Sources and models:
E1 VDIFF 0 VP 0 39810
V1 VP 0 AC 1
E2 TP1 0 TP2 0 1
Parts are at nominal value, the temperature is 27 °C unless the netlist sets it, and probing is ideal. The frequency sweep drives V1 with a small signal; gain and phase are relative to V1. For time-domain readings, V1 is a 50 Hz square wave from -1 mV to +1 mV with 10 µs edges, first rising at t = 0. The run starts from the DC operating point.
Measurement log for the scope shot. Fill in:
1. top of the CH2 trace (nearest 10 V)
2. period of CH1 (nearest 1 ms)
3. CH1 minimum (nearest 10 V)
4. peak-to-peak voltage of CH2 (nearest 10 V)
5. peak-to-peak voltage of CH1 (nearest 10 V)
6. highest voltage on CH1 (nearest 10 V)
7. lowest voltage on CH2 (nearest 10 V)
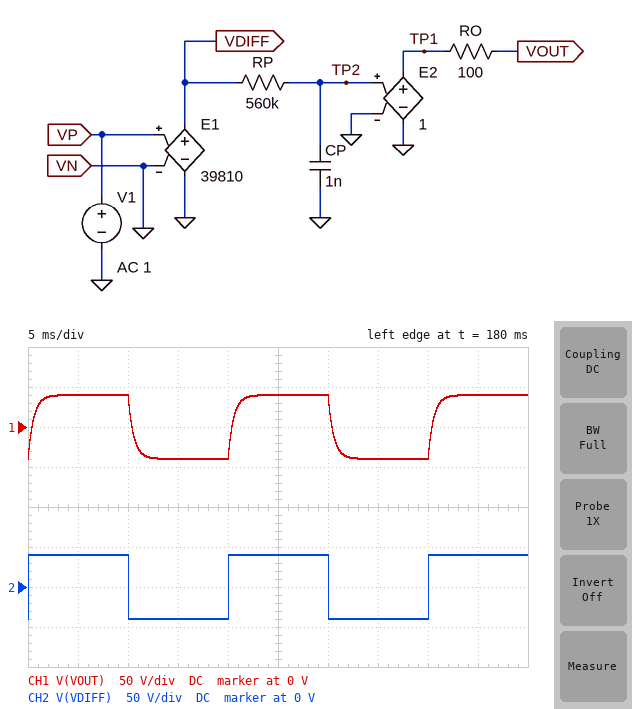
40 V
20 ms
-40 V
80 V
80 V
40 V
-40 V
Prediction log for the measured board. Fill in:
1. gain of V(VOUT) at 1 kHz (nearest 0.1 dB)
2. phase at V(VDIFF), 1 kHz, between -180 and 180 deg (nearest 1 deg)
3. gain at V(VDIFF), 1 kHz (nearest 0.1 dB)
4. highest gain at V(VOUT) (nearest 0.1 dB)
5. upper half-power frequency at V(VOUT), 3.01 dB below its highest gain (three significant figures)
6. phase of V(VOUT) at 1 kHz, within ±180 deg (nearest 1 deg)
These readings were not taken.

80.7 dB
0 deg
92.0 dB
92.0 dB
284 Hz
-74 deg
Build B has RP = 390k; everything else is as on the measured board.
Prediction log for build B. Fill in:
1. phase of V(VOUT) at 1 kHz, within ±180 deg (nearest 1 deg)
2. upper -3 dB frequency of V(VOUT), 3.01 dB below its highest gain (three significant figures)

-68 deg
408 Hz
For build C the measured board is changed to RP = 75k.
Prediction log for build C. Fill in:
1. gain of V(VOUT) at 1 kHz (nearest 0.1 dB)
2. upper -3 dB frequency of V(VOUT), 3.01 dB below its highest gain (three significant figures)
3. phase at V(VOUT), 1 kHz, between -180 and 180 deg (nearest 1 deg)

91.1 dB
2.12 kHz
-25 deg
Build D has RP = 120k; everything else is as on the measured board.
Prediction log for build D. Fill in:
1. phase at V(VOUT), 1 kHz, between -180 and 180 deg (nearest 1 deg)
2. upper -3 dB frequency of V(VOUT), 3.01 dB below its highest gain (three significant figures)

-37 deg
1.33 kHz
